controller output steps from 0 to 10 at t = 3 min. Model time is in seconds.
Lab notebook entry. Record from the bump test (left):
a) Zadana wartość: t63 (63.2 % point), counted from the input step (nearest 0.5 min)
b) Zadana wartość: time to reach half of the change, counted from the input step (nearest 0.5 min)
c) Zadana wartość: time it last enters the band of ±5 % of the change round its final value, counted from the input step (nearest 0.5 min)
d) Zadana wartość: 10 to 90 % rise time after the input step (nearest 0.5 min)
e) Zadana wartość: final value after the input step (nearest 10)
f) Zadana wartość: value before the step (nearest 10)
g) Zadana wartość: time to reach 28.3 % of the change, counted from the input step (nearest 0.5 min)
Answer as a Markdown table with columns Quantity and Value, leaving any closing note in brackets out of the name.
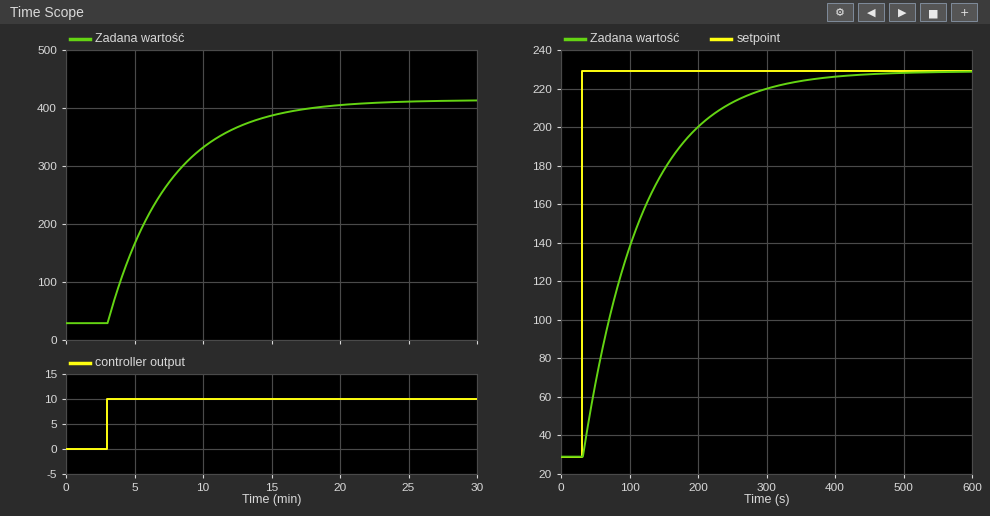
| Quantity | Value |
|---|---|
| Zadana wartość: t63 (63.2 % point), counted from the input step | 4.5 min |
| Zadana wartość: time to reach half of the change, counted from the input step | 3.0 min |
| Zadana wartość: time it last enters the band of ±5 % of the change round its final value, counted from the input step | 13.5 min |
| Zadana wartość: 10 to 90 % rise time after the input step | 10.0 min |
| Zadana wartość: final value after the input step | 410 |
| Zadana wartość: value before the step | 30 |
| Zadana wartość: time to reach 28.3 % of the change, counted from the input step | 1.5 min |
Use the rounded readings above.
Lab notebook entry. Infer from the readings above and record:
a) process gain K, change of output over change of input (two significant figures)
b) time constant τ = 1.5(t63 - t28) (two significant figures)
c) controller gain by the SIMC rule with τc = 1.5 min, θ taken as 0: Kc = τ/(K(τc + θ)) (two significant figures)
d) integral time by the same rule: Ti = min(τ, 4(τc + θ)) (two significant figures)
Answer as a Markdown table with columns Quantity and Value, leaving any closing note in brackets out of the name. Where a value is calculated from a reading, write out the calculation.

| Quantity | Value |
|---|---|
| process gain K, change of output over change of input | (410 - 30) / 10 = 38 |
| time constant τ = 1.5(t63 - t28) | 1.5 × (4.5 - 1.5) = 4.5 min |
| controller gain by the SIMC rule with τc = 1.5 min, θ taken as 0: Kc = τ/(K(τc + θ)) | 4.5 / (38 × (1.5 + 0)) = 0.079 |
| integral time by the same rule: Ti = min(τ, 4(τc + θ)) | min(4.5, 4 × (1.5 + 0)) = 4.5 min |
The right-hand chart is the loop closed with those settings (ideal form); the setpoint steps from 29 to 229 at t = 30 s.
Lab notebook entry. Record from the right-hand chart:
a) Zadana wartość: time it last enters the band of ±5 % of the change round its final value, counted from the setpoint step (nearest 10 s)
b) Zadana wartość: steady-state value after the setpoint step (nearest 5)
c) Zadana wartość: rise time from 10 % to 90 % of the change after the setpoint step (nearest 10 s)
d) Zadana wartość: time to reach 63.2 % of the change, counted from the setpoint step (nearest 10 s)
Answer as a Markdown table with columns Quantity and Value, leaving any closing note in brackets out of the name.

| Quantity | Value |
|---|---|
| Zadana wartość: time it last enters the band of ±5 % of the change round its final value, counted from the setpoint step | 260 s |
| Zadana wartość: steady-state value after the setpoint step | 230 |
| Zadana wartość: rise time from 10 % to 90 % of the change after the setpoint step | 190 s |
| Zadana wartość: time to reach 63.2 % of the change, counted from the setpoint step | 90 s |
